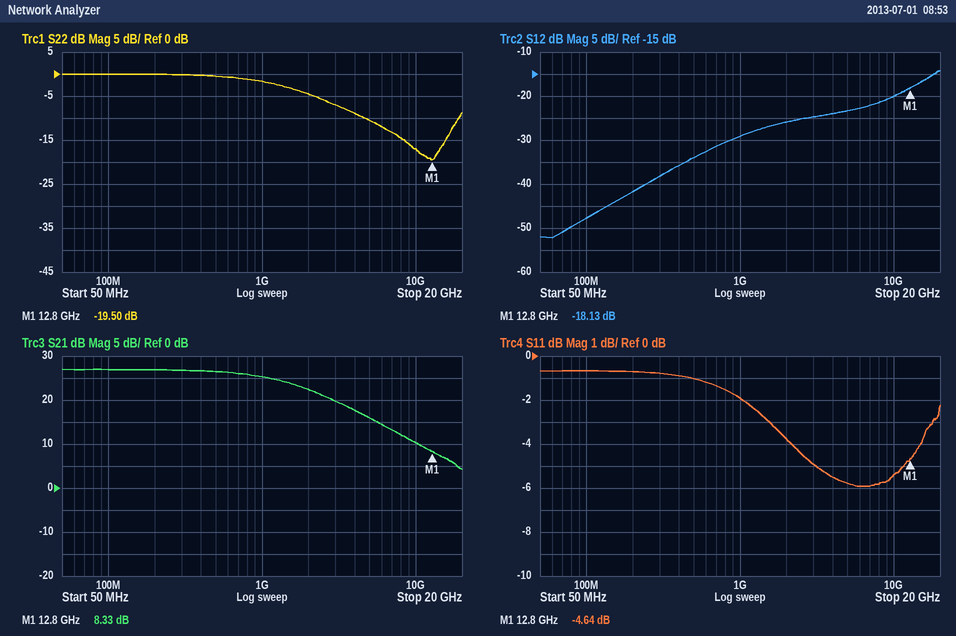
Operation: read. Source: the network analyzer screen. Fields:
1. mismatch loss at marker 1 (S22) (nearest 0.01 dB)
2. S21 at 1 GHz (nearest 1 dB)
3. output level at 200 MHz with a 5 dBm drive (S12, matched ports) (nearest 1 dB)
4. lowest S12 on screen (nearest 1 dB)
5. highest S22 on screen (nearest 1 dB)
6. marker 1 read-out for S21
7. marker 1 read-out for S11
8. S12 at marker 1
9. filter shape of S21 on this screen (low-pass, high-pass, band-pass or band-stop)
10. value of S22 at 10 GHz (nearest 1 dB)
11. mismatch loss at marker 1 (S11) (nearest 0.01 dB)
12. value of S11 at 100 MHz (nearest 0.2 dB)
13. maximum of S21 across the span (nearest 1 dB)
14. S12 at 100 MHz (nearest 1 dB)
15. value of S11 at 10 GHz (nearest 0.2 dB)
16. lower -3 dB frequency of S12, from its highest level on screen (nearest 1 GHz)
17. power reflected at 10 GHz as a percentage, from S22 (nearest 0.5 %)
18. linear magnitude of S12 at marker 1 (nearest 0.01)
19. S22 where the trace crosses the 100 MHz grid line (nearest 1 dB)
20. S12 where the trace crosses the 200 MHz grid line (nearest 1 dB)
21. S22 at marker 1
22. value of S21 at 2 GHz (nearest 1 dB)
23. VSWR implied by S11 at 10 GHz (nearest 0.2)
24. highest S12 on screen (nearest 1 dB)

0.05 dB
25 dB
-37 dBm
-52 dB
0 dB
8.33 dB
-4.64 dB
-18.13 dB
low-pass
-17 dB
1.83 dB
-0.6 dB
27 dB
-48 dB
-5.4 dB
14 GHz
2.0 %
0.12
0 dB
-42 dB
-19.50 dB
22 dB
3.4
-14 dB
